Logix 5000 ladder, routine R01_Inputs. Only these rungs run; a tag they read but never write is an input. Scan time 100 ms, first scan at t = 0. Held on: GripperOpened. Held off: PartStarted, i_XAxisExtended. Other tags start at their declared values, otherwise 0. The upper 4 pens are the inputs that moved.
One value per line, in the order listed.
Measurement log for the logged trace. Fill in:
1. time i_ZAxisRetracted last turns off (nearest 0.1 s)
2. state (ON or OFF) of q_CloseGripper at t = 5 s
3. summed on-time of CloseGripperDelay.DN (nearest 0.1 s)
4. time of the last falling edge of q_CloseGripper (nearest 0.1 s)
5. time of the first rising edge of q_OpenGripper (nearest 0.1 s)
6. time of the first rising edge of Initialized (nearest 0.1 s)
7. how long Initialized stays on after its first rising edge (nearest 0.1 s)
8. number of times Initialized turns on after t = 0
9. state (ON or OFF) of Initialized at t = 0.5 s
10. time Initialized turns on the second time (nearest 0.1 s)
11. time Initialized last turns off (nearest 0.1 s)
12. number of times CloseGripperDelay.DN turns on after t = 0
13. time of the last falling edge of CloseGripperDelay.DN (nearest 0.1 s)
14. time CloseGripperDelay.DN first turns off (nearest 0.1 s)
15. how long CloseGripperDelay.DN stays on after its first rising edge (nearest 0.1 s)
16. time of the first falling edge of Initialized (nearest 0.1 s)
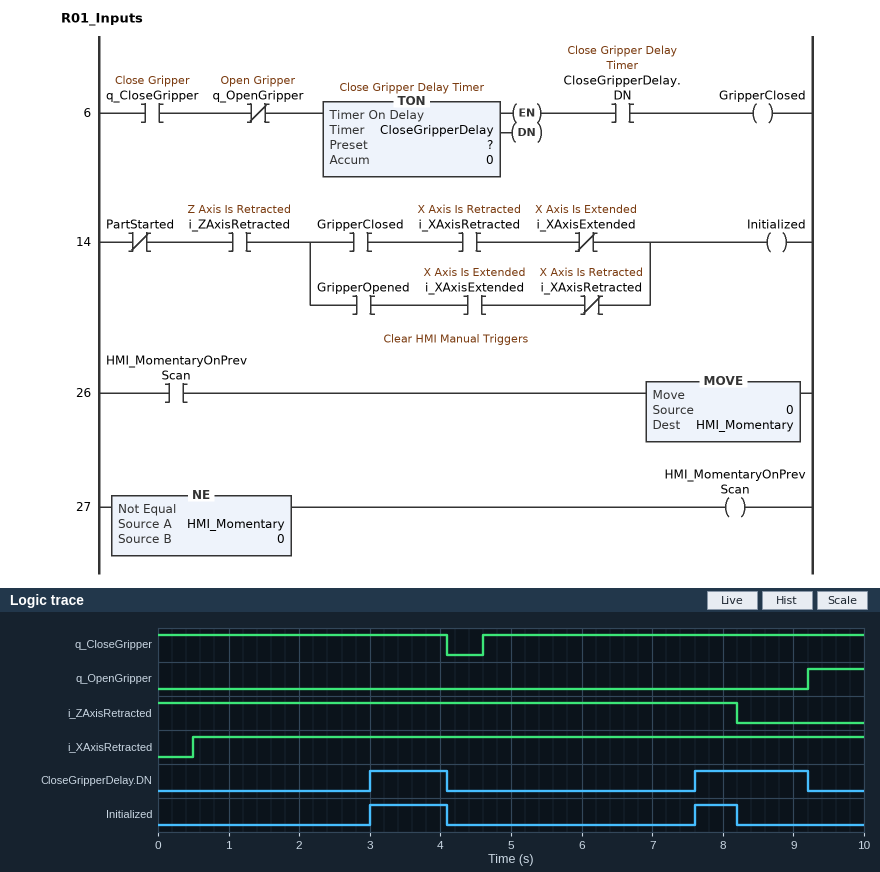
8.2 s
ON
2.7 s
4.1 s
9.2 s
3.0 s
1.1 s
2
OFF
7.6 s
8.2 s
2
9.2 s
4.1 s
1.1 s
4.1 s
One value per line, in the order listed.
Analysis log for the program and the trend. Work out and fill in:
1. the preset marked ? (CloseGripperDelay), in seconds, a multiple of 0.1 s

3.0 s
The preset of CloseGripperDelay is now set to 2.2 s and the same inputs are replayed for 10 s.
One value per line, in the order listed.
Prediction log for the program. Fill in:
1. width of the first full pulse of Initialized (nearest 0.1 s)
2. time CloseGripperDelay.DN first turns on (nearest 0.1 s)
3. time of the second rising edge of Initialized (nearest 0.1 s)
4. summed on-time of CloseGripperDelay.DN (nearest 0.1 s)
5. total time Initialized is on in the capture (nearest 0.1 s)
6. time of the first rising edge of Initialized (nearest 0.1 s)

1.9 s
2.2 s
6.8 s
4.3 s
3.3 s
2.2 s
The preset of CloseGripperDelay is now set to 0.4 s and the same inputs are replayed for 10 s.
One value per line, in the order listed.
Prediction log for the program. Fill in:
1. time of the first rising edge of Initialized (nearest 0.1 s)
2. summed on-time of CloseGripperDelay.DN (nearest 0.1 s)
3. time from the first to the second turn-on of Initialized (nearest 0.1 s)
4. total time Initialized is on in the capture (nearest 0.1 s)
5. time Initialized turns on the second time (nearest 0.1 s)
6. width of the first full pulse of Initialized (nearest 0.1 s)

0.5 s
7.9 s
4.5 s
6.8 s
5.0 s
3.6 s
